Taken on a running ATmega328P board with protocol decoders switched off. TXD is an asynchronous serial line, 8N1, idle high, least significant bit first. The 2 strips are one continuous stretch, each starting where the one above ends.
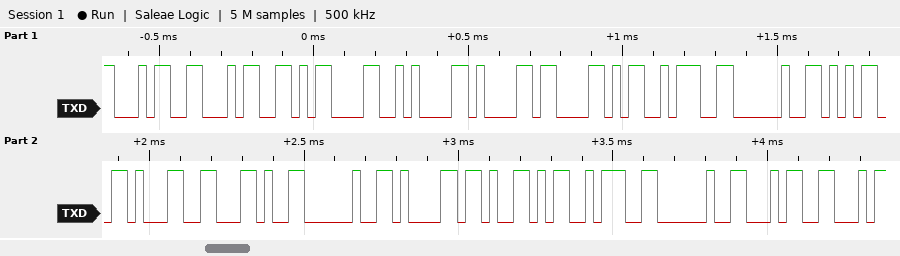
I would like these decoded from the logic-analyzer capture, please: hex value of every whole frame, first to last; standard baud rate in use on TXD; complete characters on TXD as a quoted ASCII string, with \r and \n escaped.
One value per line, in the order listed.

34 34 0D 0A 61 58 3A 20 35 31 2C 20 61 59 3A 20 34
38400 baud
"44\r\naX: 51, aY: 4"
